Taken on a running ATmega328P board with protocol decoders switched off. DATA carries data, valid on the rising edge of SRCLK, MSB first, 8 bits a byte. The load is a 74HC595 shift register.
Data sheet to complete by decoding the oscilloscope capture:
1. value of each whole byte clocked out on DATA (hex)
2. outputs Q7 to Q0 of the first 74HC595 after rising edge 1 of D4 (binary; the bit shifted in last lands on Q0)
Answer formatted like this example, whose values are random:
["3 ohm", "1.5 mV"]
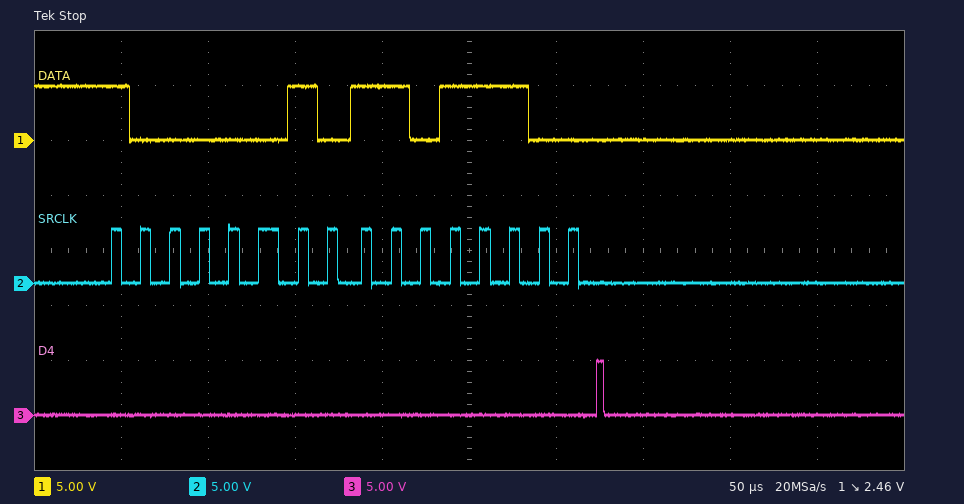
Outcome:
["0x82 0xDC", "11011100"]
